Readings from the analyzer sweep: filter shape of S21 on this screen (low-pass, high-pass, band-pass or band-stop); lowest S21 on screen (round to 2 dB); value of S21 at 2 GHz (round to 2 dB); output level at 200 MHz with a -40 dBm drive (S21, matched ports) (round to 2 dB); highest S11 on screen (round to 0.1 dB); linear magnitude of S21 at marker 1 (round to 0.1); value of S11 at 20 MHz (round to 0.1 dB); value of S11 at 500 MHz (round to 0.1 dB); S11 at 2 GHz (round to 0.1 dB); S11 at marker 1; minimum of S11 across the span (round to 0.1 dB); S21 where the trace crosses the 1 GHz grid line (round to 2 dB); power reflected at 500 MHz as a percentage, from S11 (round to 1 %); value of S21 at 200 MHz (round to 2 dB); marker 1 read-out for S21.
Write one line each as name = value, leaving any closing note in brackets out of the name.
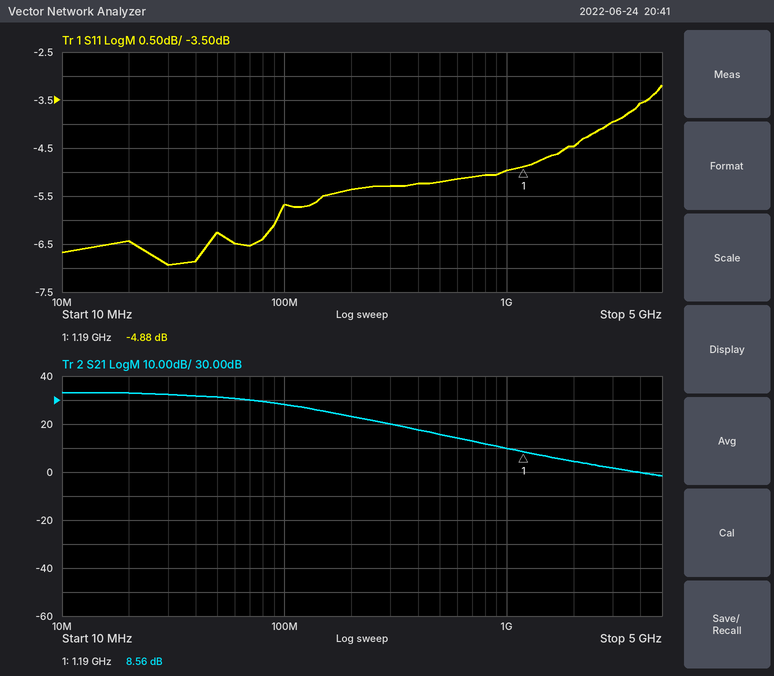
filter shape of S21 on this screen = low-pass
lowest S21 on screen = -2 dB
value of S21 at 2 GHz = 4 dB
output level at 200 MHz with a -40 dBm drive (S21, matched ports) = -16 dBm
highest S11 on screen = -3.2 dB
linear magnitude of S21 at marker 1 = 2.7
value of S11 at 20 MHz = -6.4 dB
value of S11 at 500 MHz = -5.2 dB
S11 at 2 GHz = -4.5 dB
S11 at marker 1 = -4.88 dB
minimum of S11 across the span = -6.9 dB
S21 where the trace crosses the 1 GHz grid line = 10 dB
power reflected at 500 MHz as a percentage, from S11 = 30 %
value of S21 at 200 MHz = 24 dB
marker 1 read-out for S21 = 8.56 dB
